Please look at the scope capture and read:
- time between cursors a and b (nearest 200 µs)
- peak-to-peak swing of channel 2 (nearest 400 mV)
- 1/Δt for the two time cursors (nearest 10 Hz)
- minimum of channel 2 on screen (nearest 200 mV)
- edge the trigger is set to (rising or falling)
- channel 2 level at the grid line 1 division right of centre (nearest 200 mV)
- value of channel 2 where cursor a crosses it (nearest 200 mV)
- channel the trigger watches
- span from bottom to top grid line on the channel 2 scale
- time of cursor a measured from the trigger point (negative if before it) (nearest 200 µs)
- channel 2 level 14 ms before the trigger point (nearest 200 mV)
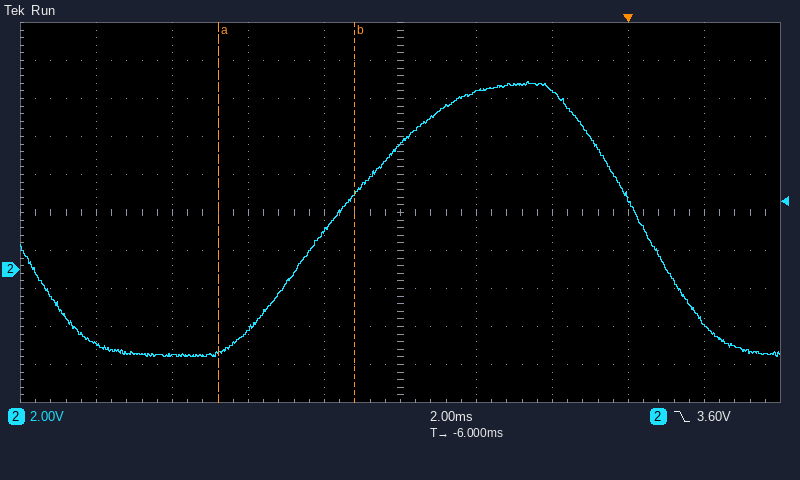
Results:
3.6 ms
14.4 V
280 Hz
-4.6 V
falling
9.4 V
-4.4 V
channel 2
20 V
-10.8 ms
-4.0 V
